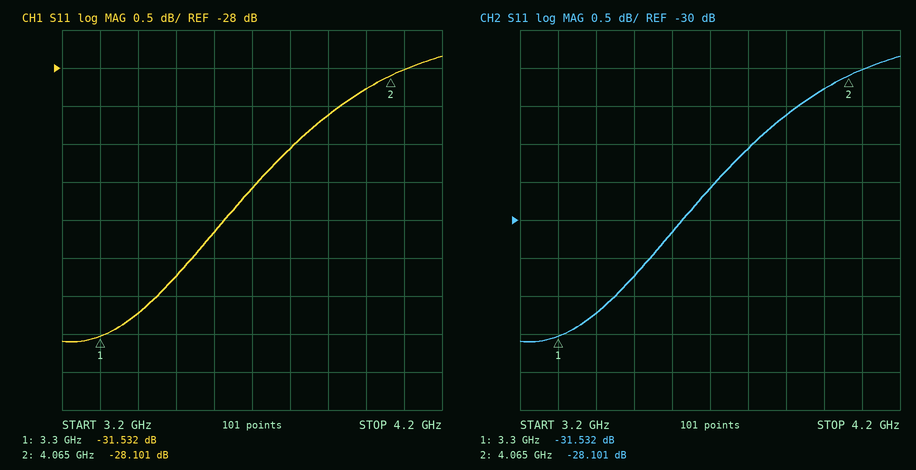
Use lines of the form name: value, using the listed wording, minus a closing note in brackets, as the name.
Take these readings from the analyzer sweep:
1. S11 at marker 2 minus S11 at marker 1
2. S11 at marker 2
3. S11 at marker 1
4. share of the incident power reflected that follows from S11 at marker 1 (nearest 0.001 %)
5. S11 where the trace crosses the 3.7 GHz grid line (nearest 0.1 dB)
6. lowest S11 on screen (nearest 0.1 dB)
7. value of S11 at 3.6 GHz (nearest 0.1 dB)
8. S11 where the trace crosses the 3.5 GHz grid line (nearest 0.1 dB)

S11 at marker 2 minus S11 at marker 1: 3.431 dB
S11 at marker 2: -28.101 dB
S11 at marker 1: -31.532 dB
share of the incident power reflected that follows from S11 at marker 1: 0.070 %
S11 where the trace crosses the 3.7 GHz grid line: -29.6 dB
lowest S11 on screen: -31.6 dB
value of S11 at 3.6 GHz: -30.2 dB
S11 where the trace crosses the 3.5 GHz grid line: -30.7 dB
